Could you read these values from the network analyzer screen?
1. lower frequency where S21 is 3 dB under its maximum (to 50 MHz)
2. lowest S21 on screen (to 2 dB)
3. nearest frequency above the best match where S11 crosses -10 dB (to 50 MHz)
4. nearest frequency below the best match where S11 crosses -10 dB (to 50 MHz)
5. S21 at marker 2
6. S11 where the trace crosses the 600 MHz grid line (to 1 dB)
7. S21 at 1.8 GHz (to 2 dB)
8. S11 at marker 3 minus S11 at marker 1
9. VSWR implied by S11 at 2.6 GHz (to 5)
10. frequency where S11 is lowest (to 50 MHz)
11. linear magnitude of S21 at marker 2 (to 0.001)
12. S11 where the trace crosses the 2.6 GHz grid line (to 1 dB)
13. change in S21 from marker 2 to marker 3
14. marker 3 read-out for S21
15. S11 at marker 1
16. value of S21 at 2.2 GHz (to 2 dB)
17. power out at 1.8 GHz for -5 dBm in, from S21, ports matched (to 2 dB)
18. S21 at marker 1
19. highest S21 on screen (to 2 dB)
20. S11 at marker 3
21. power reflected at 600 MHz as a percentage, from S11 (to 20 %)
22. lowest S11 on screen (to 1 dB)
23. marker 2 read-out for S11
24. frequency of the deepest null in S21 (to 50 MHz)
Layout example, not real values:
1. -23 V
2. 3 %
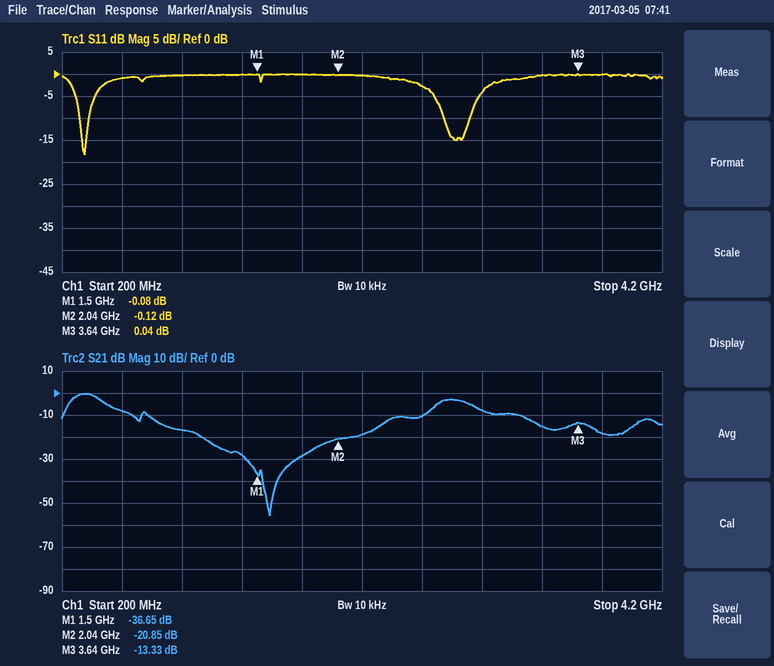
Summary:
1. 250 MHz
2. -56 dB
3. 400 MHz
4. 300 MHz
5. -20.85 dB
6. -1 dB
7. -28 dB
8. 0.12 dB
9. 5
10. 350 MHz
11. 0.091
12. -3 dB
13. 7.52 dB
14. -13.33 dB
15. -0.08 dB
16. -18 dB
17. -34 dBm
18. -36.65 dB
19. 0 dB
20. 0.04 dB
21. 80 %
22. -18 dB
23. -0.12 dB
24. 1.60 GHz
